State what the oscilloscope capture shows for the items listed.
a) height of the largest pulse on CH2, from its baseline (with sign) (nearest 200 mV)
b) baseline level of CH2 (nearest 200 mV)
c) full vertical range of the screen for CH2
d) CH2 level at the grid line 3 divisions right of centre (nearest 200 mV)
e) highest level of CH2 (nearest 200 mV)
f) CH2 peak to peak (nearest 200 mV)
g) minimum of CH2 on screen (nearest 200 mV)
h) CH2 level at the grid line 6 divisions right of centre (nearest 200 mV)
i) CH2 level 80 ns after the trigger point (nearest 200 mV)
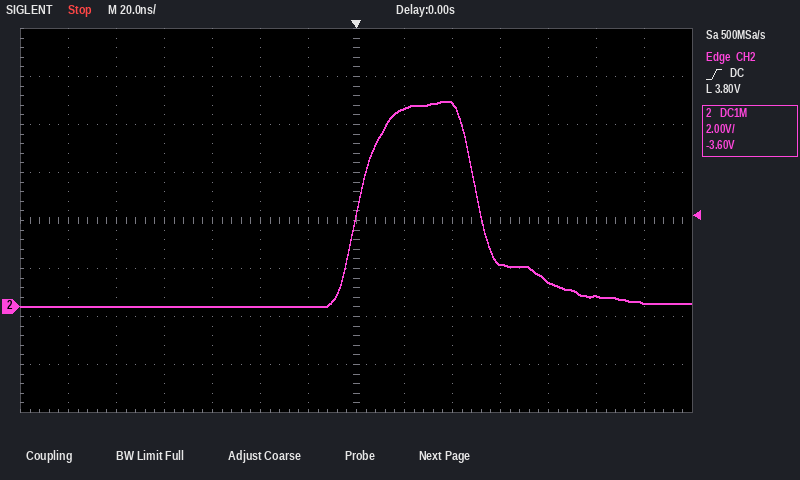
+8.6 V
0.0 V
16 V
1.8 V
8.6 V
8.6 V
0.0 V
200 mV
1.0 V
